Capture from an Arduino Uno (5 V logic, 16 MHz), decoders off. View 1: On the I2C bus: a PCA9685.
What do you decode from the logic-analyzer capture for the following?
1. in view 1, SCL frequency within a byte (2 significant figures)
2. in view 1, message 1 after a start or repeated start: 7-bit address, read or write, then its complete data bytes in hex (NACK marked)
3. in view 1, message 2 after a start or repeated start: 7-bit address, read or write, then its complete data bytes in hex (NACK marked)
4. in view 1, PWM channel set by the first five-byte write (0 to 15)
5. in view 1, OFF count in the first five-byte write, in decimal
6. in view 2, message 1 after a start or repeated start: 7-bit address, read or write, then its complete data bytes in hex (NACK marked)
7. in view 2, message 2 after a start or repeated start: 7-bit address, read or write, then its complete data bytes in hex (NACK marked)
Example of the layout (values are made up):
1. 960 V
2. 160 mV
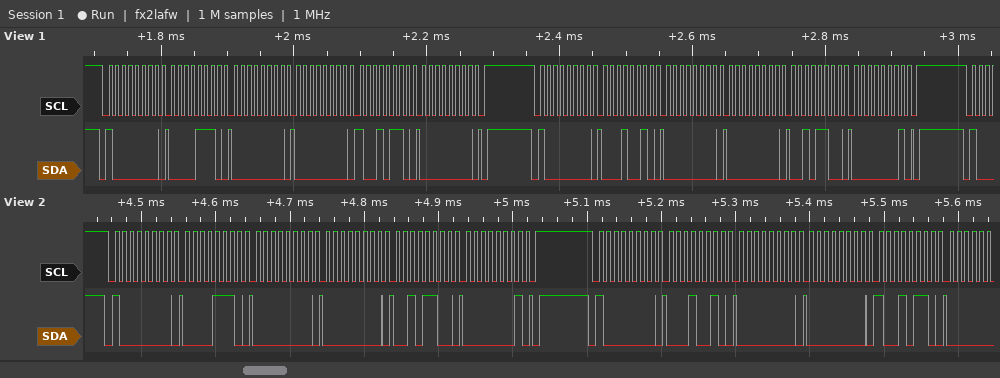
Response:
1. 100 kHz
2. 0x40 write: 0E 00 00 96 00
3. 0x40 write: 12 00 00 2C 01
4. 2
5. 150
6. 0x40 write: 0E 00 00 2C 01
7. 0x40 write: 12 00 00 96
